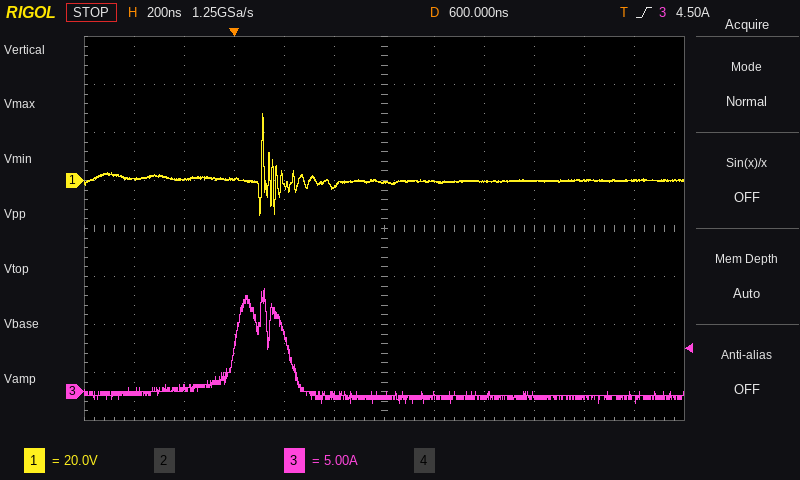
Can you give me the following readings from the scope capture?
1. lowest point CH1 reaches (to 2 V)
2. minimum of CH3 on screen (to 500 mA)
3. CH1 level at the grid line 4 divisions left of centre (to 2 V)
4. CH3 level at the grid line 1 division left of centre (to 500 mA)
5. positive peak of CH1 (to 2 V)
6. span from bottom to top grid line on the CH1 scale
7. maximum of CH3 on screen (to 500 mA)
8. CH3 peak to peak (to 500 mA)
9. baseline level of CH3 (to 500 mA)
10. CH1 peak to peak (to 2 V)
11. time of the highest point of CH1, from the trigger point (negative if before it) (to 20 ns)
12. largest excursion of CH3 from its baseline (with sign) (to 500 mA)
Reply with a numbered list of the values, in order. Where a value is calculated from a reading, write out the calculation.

1. -14 V
2. -1.0 A
3. 0 V
4. -500 mA
5. 28 V
6. 160 V
7. 11.0 A
8. 11.0 A − (-1.0 A) = 12.0 A
9. -500 mA
10. 28 V − (-14 V) = 42 V
11. +120 ns
12. 11.0 A − (-500 mA) = +11.5 A
